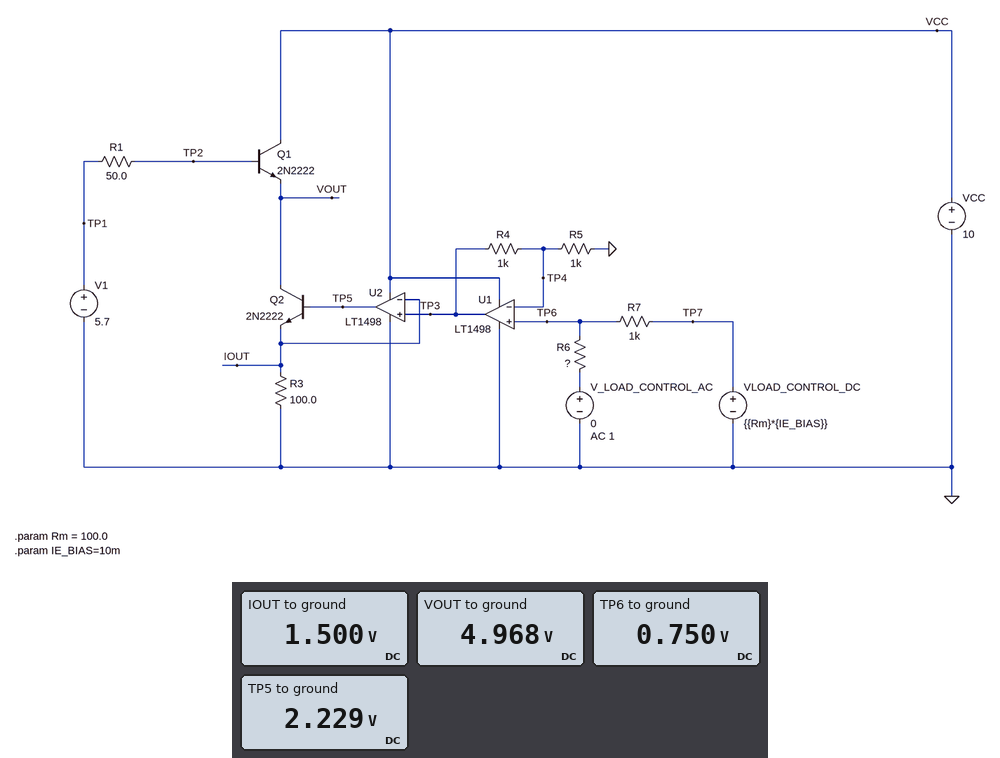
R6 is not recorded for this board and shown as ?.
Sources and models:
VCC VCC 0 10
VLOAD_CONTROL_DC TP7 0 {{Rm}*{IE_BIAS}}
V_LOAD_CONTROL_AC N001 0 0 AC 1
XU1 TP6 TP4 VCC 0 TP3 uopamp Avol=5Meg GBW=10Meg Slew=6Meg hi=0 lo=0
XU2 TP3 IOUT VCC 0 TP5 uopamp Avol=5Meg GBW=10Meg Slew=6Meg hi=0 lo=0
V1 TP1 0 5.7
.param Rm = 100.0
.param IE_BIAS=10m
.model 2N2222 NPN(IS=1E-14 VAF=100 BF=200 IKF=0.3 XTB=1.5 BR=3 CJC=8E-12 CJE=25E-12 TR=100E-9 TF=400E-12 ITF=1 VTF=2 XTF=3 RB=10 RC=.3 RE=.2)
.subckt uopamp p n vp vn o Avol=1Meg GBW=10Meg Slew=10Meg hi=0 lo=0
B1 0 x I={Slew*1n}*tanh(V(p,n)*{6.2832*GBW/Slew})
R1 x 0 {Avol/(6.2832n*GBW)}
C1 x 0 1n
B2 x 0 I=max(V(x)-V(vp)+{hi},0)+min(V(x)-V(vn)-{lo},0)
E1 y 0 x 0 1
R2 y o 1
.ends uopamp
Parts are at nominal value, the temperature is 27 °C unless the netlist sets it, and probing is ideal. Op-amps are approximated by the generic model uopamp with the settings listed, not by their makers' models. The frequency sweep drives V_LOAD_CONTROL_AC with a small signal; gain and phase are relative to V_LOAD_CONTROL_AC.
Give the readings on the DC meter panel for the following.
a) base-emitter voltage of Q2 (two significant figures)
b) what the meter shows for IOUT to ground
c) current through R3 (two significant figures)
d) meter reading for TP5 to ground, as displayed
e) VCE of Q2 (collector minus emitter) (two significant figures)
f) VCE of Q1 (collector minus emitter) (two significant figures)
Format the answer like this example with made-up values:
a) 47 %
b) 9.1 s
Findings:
a) 730 mV
b) 1.500 V
c) 15 mA
d) 2.229 V
e) 3.5 V
f) 5.0 V
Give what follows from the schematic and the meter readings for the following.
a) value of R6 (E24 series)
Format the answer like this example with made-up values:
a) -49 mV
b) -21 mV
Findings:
a) 3 kΩ
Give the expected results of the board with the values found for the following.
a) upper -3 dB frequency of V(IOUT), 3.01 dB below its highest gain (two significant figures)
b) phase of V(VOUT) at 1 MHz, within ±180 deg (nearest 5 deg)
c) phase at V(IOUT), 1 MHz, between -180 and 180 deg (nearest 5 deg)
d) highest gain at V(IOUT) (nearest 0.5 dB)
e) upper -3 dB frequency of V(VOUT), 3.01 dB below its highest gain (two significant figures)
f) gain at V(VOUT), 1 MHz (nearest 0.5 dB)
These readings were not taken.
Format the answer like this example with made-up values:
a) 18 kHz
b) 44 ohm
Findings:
a) 4.2 MHz
b) 165 deg
c) -15 deg
d) -6.0 dB
e) 4.6 MHz
f) -39.0 dB
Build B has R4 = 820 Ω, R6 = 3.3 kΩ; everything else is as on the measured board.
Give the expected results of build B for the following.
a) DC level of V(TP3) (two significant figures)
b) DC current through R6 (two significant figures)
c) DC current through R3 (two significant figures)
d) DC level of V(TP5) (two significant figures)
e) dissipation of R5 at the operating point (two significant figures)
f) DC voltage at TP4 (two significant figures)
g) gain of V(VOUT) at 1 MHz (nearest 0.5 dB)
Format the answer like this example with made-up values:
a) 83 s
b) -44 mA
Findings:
a) 1.4 V
b) 230 µA
c) 14 mA
d) 2.1 V
e) 590 µW
f) 770 mV
g) -40.0 dB
